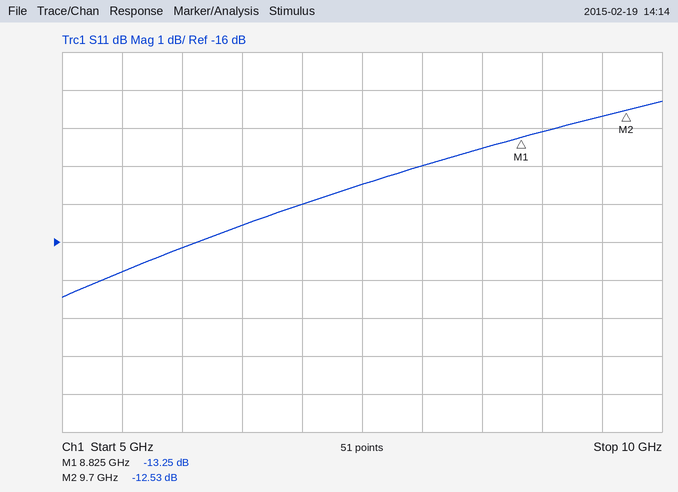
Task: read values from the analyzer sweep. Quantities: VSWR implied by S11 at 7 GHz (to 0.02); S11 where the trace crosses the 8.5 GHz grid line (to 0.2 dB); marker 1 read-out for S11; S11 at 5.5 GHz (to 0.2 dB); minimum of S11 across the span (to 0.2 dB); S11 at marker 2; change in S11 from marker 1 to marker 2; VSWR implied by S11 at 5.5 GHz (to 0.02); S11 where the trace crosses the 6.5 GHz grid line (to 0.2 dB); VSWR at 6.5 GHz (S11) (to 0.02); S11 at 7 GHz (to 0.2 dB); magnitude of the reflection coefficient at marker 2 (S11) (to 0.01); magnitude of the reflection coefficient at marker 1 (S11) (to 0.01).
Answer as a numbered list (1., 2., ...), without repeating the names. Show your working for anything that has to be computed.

1. |Γ| = 10^(-15/20) = 0.1778; VSWR = (1 + 0.1778)/(1 − 0.1778) ≈ 1.43, so 1.44 to the nearest 0.02
2. -13.6 dB
3. -13.25 dB
4. -16.8 dB
5. -17.4 dB
6. -12.53 dB
7. -12.53 − (-13.25) = 0.72 dB
8. |Γ| = 10^(-16.8/20) = 0.1445; VSWR = (1 + 0.1445)/(1 − 0.1445) ≈ 1.34
9. -15.6 dB
10. |Γ| = 10^(-15.6/20) = 0.1660; VSWR = (1 + 0.1660)/(1 − 0.1660) ≈ 1.40
11. -15.0 dB
12. 10^(-12.53/20) ≈ 0.24
13. 10^(-13.25/20) ≈ 0.22
